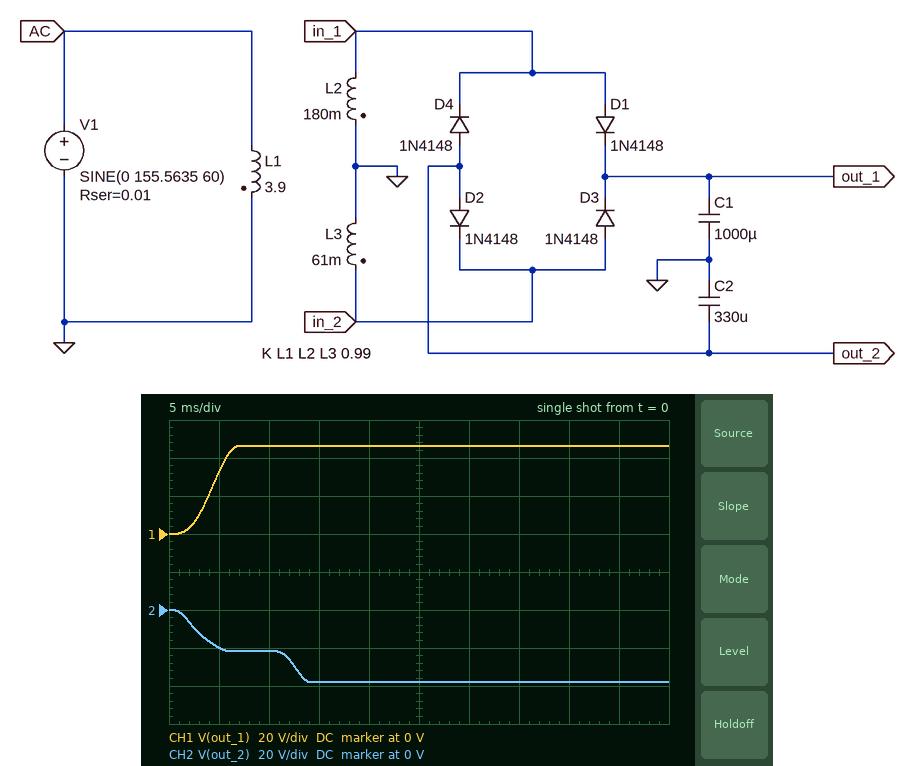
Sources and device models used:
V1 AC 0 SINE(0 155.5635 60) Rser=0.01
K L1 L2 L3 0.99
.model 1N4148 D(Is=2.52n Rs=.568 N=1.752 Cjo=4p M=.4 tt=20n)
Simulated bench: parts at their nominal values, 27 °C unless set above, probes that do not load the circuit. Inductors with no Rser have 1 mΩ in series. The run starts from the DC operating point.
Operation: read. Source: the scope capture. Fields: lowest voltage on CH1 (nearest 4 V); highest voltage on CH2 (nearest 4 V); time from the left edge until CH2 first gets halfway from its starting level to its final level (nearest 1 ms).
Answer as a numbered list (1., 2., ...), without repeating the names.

1. 0 V
2. 0 V
3. 5 ms
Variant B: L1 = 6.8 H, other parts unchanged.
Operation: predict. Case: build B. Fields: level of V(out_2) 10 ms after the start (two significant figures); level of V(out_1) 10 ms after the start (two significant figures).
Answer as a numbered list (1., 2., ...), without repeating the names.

1. -16 V
2. 35 V
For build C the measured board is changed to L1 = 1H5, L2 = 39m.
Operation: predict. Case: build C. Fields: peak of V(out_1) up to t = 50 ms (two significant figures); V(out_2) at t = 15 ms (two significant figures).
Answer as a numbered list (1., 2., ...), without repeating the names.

1. 30 V
2. -37 V
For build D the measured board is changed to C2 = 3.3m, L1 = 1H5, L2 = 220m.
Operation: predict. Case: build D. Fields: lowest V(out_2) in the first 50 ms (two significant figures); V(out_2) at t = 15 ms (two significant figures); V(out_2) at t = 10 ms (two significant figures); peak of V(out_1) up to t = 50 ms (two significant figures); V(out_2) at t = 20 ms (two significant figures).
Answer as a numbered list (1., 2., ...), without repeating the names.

1. -52 V
2. -43 V
3. -30 V
4. 79 V
5. -46 V
